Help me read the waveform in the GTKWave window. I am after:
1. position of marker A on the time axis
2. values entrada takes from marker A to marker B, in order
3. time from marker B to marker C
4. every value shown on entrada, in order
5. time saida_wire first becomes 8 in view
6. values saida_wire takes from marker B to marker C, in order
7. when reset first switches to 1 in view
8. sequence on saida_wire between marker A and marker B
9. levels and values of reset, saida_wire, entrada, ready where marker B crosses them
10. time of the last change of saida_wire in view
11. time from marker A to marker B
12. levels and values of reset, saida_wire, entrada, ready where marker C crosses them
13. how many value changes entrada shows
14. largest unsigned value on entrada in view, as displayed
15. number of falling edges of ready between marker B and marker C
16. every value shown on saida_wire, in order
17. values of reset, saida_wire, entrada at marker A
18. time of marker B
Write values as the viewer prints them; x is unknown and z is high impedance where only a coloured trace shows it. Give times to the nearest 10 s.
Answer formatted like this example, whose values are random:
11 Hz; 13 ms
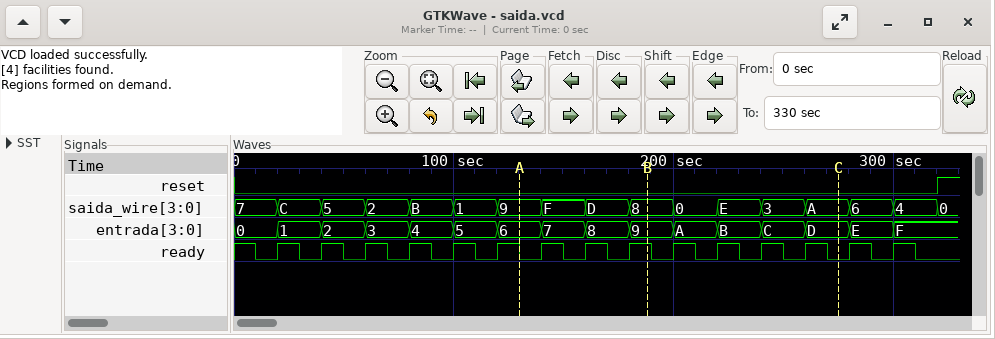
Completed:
130 s; 6, 7, 8, 9; 90 s; 0, 1, 2, 3, 4, 5, 6, 7, 8, 9, A, B, C, D, E, F; 180 s; 8, 0, E, 3, A; 320 s; 9, F, D, 8; reset=0, saida_wire=8, entrada=9, ready=1; 320 s; 60 s; reset=0, saida_wire=A, entrada=D, ready=0; 15; F; 5; 7, C, 5, 2, B, 1, 9, F, D, 8, 0, E, 3, A, 6, 4, 0; reset=0, saida_wire=9, entrada=6; 190 s
